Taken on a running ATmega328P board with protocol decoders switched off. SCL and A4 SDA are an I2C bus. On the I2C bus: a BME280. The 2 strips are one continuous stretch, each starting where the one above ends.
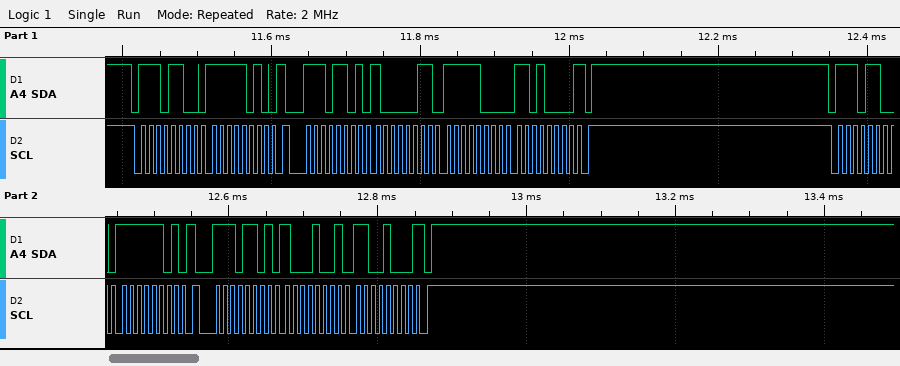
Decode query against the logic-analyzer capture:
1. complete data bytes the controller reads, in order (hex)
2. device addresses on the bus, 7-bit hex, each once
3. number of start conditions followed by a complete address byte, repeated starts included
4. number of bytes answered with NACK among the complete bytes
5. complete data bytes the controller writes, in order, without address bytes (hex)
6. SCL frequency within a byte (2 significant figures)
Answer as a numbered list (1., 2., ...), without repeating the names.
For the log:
1. 83 F8 D0 89 C8
2. 0x76
3. 4
4. 2
5. FA FD
6. 100 kHz
